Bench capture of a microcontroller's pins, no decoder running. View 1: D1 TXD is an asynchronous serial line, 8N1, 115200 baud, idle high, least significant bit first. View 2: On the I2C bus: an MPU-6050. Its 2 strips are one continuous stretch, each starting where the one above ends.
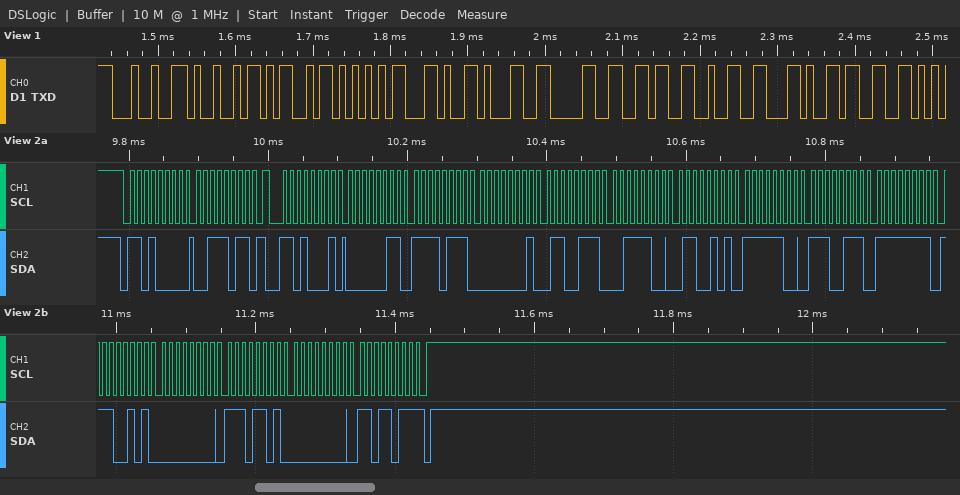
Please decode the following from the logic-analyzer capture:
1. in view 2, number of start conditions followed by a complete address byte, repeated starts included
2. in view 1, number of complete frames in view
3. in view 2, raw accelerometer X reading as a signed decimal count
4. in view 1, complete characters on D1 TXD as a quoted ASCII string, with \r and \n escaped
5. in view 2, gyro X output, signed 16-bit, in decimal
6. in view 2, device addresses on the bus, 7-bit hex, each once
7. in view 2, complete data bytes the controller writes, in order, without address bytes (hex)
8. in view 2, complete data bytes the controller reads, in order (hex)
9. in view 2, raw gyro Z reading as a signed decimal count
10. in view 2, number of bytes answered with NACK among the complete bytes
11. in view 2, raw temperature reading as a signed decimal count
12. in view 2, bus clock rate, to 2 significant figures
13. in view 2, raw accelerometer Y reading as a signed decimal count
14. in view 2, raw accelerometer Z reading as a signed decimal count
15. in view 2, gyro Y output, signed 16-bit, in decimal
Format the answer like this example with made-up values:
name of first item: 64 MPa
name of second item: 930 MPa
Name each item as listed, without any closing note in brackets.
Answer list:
in view 2, number of start conditions followed by a complete address byte, repeated starts included: 2
in view 1, number of complete frames in view: 11
in view 2, raw accelerometer X reading as a signed decimal count: 1015
in view 1, complete characters on D1 TXD as a quoted ASCII string, with \r and \n escaped: "$IMU,1062,3"
in view 2, gyro X output, signed 16-bit, in decimal: -27
in view 2, device addresses on the bus, 7-bit hex, each once: 0x68
in view 2, complete data bytes the controller writes, in order, without address bytes: 3B
in view 2, complete data bytes the controller reads, in order: 03 F7 01 67 3C 65 FC E7 FF E5 00 ED 00 DB
in view 2, raw gyro Z reading as a signed decimal count: 219
in view 2, number of bytes answered with NACK among the complete bytes: 1
in view 2, raw temperature reading as a signed decimal count: -793
in view 2, bus clock rate, to 2 significant figures: 100 kHz
in view 2, raw accelerometer Y reading as a signed decimal count: 359
in view 2, raw accelerometer Z reading as a signed decimal count: 15461
in view 2, gyro Y output, signed 16-bit, in decimal: 237
